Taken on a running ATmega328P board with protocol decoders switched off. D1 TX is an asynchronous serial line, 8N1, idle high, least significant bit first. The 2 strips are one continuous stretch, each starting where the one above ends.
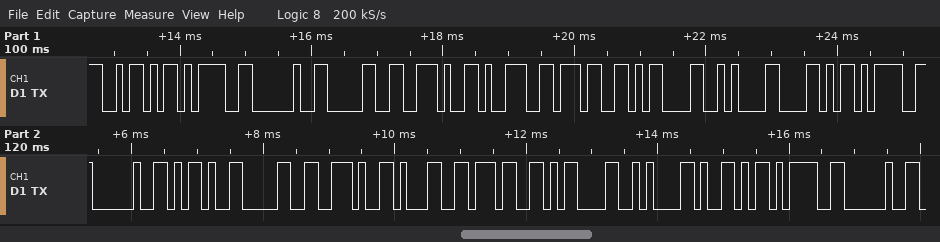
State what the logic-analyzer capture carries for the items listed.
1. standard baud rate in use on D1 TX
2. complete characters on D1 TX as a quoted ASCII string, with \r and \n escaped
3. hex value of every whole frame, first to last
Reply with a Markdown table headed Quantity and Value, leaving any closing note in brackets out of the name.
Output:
| Quantity | Value |
|---|---|
| standard baud rate in use on D1 TX | 9600 baud |
| complete characters on D1 TX as a quoted ASCII string, with \r and \n escaped | "Z= 0.97\r\nX= -0.17\r\nY= " |
| hex value of every whole frame, first to last | 5A 3D 20 30 2E 39 37 0D 0A 58 3D 20 2D 30 2E 31 37 0D 0A 59 3D 20 |
